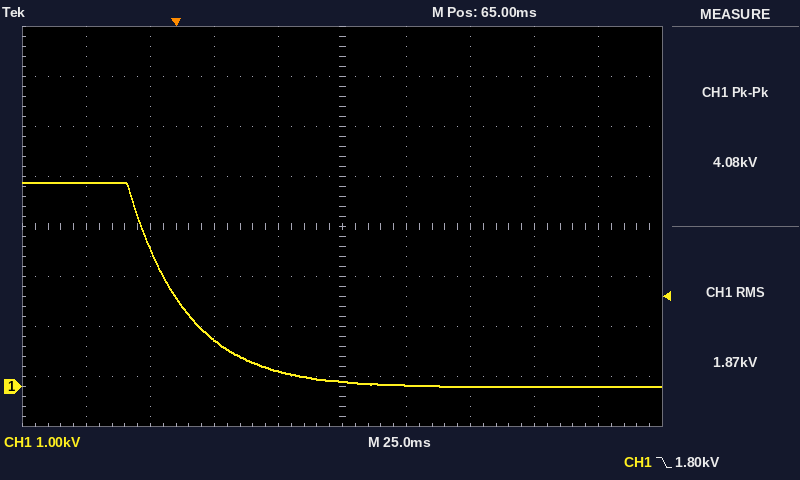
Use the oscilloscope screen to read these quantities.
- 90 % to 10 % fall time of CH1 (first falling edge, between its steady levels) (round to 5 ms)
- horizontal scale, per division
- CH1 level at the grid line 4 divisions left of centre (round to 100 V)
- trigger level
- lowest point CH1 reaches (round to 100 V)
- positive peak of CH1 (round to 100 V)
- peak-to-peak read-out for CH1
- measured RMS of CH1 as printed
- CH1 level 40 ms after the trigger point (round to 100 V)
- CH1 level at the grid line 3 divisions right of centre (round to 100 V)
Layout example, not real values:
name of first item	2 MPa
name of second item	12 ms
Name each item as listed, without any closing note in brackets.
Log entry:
90 % to 10 % fall time of CH1 (first falling edge, between its steady levels)	50 ms
horizontal scale, per division	25 ms
CH1 level at the grid line 4 divisions left of centre	4.1 kV
trigger level	1.80 kV
lowest point CH1 reaches	0.0 kV
positive peak of CH1	4.1 kV
peak-to-peak read-out for CH1	4.08 kV
measured RMS of CH1 as printed	1.87 kV
CH1 level 40 ms after the trigger point	300 V
CH1 level at the grid line 3 divisions right of centre	0.0 kV
